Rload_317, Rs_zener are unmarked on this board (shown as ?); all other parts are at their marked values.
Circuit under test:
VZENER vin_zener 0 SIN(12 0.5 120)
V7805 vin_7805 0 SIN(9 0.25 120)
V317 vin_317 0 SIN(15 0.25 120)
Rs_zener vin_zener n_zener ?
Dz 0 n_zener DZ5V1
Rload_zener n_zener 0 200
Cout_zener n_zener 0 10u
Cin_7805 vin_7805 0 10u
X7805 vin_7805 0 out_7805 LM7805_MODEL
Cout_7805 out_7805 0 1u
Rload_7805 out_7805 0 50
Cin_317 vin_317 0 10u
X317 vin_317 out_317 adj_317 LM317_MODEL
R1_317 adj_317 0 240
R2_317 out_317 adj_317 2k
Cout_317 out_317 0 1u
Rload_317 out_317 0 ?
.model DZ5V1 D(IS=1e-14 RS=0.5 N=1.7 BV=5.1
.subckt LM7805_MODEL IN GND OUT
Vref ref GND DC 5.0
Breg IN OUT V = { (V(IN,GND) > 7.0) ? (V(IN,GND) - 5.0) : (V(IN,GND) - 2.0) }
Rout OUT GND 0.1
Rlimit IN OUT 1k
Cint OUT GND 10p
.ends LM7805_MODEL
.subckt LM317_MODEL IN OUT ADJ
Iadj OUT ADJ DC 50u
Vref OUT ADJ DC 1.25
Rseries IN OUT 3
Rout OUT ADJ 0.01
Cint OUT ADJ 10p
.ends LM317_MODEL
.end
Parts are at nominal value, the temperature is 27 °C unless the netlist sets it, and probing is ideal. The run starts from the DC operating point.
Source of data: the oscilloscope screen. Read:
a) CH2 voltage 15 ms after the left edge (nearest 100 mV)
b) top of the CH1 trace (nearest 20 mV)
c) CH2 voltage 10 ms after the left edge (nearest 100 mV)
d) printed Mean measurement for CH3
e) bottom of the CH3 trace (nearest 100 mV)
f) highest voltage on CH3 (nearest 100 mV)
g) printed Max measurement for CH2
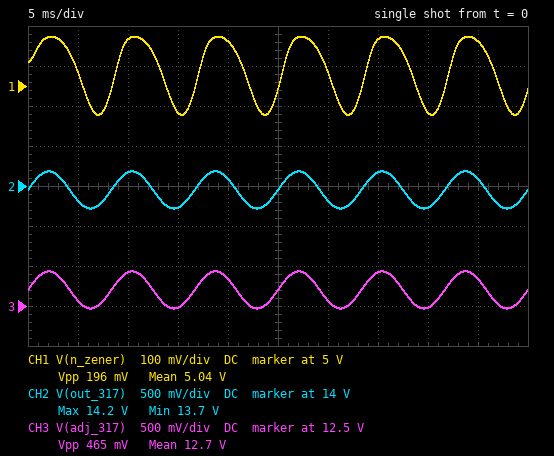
13.7 V
5.12 V
14.2 V
12.7 V
12.5 V
12.9 V
14.2 V
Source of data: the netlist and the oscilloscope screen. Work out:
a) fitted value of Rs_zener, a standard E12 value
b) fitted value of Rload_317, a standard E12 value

270 Ω
47 Ω
